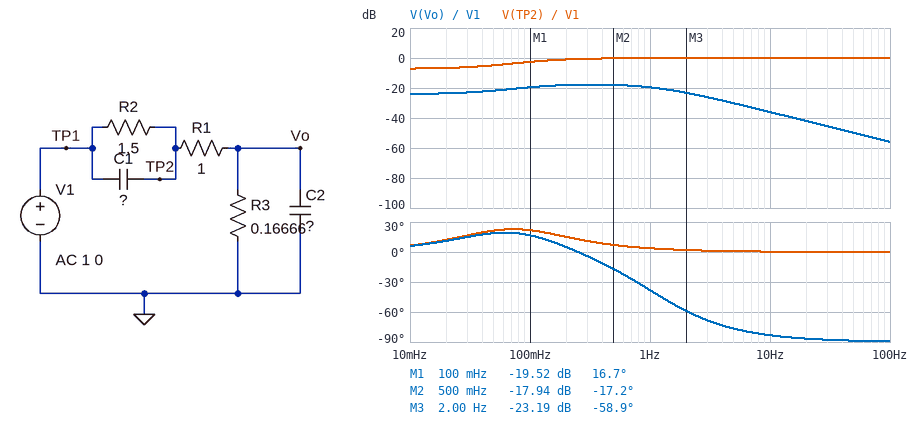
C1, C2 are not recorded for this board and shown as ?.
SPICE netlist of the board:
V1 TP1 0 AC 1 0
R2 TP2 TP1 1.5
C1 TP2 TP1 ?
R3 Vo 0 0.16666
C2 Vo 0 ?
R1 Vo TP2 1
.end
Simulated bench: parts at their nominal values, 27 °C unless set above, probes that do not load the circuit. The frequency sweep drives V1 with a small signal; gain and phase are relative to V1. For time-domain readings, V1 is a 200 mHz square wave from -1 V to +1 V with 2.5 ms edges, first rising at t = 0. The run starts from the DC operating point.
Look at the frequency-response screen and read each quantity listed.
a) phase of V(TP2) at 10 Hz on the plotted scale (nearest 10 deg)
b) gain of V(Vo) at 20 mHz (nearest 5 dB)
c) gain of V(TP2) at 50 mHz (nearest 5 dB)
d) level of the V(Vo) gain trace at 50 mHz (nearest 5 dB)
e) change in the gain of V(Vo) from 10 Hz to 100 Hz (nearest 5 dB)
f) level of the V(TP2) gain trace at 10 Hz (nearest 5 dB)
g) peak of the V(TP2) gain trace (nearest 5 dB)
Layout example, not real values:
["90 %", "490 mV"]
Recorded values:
["0 deg", "-25 dB", "-5 dB", "-20 dB", "-20 dB", "0 dB", "0 dB"]
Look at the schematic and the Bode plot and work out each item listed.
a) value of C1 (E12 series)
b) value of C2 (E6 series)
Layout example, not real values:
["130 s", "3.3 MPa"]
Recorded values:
["2.2 F", "1 F"]
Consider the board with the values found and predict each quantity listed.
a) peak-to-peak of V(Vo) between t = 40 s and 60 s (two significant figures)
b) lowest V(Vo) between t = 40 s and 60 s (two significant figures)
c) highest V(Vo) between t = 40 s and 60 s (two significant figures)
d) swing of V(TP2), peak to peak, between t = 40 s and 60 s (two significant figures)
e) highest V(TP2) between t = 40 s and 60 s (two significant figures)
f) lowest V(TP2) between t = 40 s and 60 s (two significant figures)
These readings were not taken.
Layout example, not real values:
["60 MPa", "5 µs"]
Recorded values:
["320 mV", "-160 mV", "160 mV", "2.8 V", "1.4 V", "-1.4 V"]
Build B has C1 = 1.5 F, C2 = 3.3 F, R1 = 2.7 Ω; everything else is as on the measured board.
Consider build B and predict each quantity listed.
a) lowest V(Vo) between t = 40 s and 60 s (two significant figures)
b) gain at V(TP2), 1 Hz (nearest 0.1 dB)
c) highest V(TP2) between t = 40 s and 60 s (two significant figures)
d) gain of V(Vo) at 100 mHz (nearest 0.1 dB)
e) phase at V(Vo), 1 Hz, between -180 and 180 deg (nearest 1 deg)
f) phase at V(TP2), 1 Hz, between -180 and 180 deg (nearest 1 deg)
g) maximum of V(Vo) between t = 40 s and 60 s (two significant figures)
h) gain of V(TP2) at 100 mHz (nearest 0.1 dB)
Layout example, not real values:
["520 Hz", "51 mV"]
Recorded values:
["-49 mV", "0 dB", "1.2 V", "-26.8 dB", "-71 deg", "2 deg", "49 mV", "-1.6 dB"]
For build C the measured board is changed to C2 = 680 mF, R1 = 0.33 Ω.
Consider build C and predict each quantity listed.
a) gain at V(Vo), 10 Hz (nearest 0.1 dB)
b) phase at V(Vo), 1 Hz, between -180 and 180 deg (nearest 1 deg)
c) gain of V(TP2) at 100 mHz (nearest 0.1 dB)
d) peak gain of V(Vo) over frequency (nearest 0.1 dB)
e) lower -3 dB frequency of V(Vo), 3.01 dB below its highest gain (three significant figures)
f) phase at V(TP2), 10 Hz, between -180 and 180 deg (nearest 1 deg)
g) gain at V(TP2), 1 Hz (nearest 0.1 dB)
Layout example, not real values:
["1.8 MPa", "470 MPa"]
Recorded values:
["-23.2 dB", "-17 deg", "-5.9 dB", "-10.5 dB", "149 mHz", "1 deg", "-0.4 dB"]
